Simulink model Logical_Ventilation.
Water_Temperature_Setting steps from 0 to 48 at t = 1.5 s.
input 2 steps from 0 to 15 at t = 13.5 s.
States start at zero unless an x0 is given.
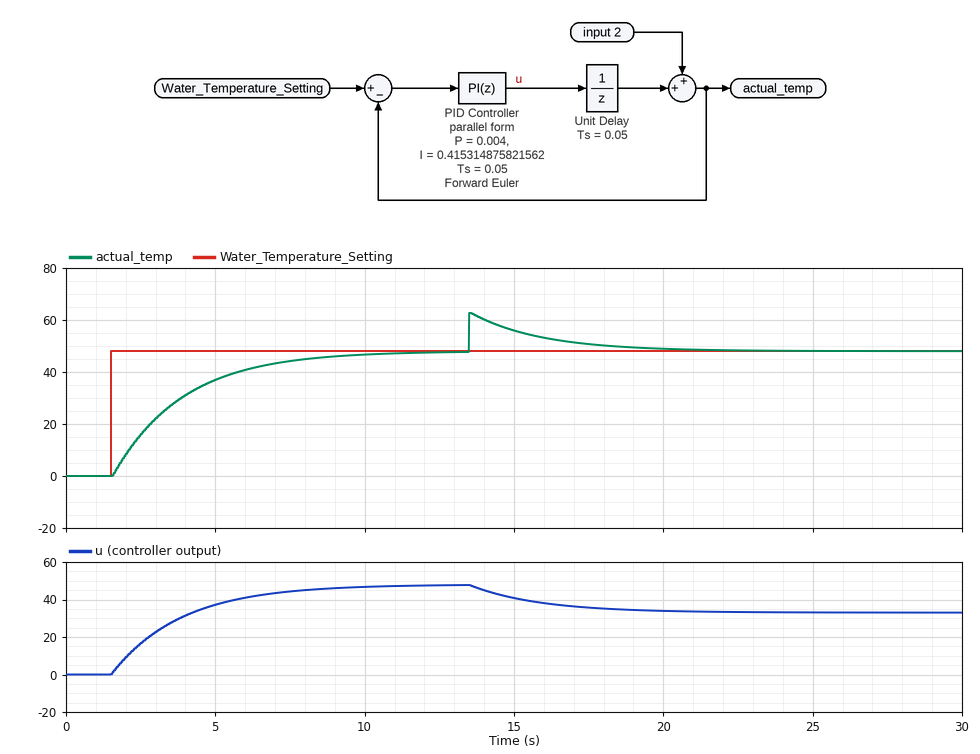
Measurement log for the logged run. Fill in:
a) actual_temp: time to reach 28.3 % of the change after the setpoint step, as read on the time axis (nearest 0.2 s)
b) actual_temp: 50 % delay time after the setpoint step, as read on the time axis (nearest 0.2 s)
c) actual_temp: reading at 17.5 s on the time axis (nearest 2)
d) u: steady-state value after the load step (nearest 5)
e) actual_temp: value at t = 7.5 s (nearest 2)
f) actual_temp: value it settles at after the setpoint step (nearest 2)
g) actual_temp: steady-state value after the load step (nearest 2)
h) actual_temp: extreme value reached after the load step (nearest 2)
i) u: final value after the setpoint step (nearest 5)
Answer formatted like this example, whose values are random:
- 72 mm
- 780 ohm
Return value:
- 2.4 s
- 3.2 s
- 50
- 35
- 44
- 48
- 48
- 62
- 50
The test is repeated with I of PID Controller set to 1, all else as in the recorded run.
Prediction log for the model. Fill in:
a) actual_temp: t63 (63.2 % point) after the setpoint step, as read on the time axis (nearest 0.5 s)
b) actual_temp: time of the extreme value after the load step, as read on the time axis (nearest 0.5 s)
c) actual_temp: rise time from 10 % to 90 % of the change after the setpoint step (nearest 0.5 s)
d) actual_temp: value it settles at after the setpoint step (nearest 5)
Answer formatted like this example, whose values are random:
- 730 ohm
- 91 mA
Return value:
- 2.5 s
- 13.5 s
- 2.0 s
- 50
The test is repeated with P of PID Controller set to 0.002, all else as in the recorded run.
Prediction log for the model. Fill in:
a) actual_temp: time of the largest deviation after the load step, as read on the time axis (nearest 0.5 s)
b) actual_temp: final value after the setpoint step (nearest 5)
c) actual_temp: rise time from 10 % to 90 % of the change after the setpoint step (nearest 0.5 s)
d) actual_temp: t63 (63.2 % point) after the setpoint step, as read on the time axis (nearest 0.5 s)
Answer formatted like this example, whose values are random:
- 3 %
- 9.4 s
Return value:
- 13.5 s
- 50
- 5.0 s
- 4.0 s
